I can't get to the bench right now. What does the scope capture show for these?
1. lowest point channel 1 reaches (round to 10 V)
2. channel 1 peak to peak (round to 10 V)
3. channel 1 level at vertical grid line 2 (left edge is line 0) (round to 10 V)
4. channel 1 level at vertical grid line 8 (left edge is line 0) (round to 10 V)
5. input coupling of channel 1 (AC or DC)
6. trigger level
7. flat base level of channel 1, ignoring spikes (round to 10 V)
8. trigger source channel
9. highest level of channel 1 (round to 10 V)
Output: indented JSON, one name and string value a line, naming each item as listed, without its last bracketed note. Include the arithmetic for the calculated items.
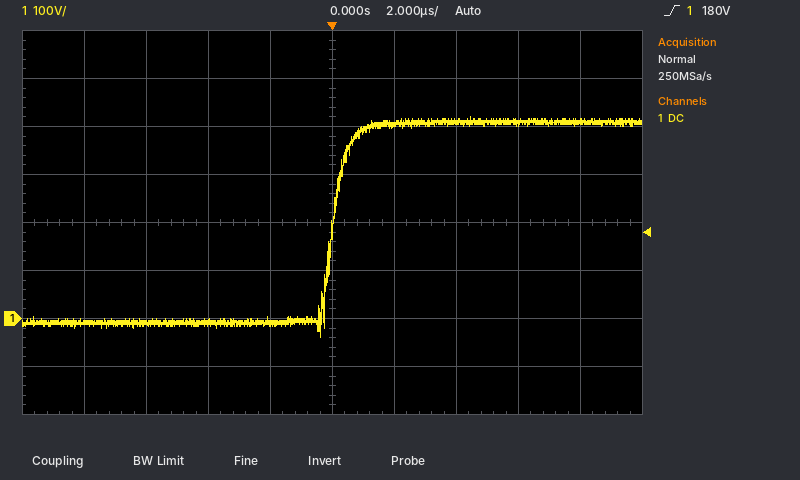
{
  "lowest point channel 1 reaches": "-40 V",
  "channel 1 peak to peak": "420 V − (-40 V) = 460 V",
  "channel 1 level at vertical grid line 2 (left edge is line 0)": "-10 V",
  "channel 1 level at vertical grid line 8 (left edge is line 0)": "410 V",
  "input coupling of channel 1": "DC",
  "trigger level": "180 V",
  "flat base level of channel 1, ignoring spikes": "-10 V",
  "trigger source channel": "channel 1",
  "highest level of channel 1": "420 V"
}
